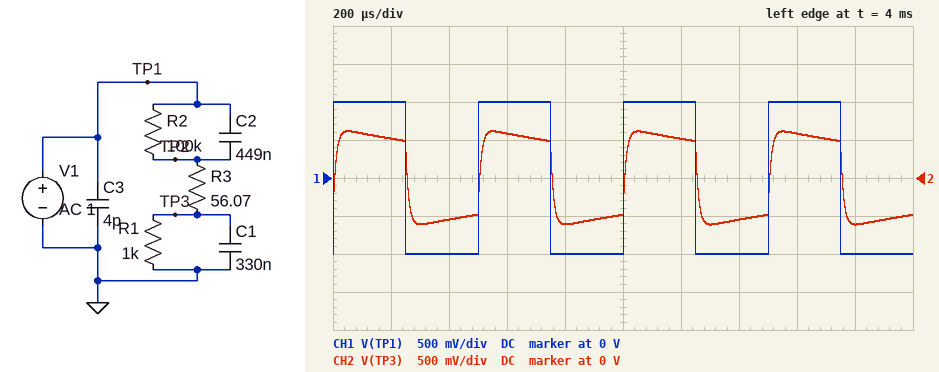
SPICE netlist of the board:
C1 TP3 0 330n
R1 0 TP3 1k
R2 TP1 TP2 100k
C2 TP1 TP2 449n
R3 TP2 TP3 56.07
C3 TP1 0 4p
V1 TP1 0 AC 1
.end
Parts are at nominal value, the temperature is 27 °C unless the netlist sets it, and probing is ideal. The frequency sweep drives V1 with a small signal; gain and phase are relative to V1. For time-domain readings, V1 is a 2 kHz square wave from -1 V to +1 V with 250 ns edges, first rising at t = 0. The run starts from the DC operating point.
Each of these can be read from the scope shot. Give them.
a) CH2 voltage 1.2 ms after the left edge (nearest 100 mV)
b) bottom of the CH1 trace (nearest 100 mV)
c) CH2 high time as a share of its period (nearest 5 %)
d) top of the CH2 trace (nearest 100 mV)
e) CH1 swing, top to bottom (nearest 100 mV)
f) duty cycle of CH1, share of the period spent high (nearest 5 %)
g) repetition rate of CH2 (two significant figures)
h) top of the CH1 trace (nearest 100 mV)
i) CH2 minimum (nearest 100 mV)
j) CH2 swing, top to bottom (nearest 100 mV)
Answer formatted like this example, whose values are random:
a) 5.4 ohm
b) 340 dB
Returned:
a) 500 mV
b) -1.0 V
c) 50 %
d) 600 mV
e) 2.0 V
f) 50 %
g) 2.0 kHz
h) 1.0 V
i) -600 mV
j) 1.2 V
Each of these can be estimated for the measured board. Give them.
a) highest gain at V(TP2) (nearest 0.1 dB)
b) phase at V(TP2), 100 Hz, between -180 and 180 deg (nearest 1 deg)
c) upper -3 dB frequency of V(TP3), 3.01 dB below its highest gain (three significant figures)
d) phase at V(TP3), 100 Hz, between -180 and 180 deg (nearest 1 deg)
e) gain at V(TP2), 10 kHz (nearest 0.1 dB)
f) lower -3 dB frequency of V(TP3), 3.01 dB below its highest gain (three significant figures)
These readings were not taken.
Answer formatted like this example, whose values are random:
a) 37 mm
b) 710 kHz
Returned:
a) 0 dB
b) 62 deg
c) 15.6 kHz
d) 61 deg
e) -2.6 dB
f) 197 Hz
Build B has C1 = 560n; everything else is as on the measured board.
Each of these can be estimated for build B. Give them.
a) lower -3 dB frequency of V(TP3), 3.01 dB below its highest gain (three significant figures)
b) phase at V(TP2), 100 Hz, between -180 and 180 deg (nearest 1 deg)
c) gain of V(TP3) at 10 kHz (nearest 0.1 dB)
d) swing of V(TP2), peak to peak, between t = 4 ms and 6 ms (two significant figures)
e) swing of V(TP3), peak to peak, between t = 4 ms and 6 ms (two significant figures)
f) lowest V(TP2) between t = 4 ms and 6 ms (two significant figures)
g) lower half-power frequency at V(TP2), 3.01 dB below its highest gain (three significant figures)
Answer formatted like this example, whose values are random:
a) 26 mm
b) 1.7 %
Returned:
a) 153 Hz
b) 56 deg
c) -9.6 dB
d) 3.2 V
e) 930 mV
f) -1.6 V
g) 8.69 kHz
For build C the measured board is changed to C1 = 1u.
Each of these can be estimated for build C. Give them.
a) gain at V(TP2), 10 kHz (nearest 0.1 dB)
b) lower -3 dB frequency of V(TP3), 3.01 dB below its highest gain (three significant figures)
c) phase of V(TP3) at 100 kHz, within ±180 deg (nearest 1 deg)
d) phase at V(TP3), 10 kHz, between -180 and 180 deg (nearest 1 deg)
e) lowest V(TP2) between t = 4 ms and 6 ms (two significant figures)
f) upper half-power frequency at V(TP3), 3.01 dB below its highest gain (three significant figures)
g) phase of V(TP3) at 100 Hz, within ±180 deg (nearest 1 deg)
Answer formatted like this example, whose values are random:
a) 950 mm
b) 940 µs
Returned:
a) -2.3 dB
b) 108 Hz
c) -85 deg
d) -47 deg
e) -1.7 V
f) 9.43 kHz
g) 45 deg
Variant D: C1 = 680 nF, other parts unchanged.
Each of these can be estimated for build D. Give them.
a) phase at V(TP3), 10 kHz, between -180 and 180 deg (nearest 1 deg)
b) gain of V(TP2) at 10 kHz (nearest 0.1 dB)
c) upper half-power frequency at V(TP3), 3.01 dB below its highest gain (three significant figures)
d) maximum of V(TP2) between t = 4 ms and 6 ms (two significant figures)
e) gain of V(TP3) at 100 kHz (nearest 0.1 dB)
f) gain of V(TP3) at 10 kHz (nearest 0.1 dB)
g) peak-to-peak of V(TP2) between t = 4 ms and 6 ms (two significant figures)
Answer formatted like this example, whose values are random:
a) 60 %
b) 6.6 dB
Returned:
a) -43 deg
b) -2.5 dB
c) 10.9 kHz
d) 1.6 V
e) -27.6 dB
f) -10.9 dB
g) 3.3 V
